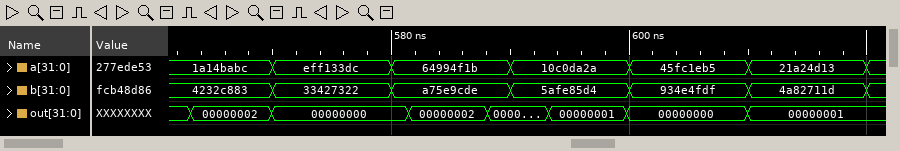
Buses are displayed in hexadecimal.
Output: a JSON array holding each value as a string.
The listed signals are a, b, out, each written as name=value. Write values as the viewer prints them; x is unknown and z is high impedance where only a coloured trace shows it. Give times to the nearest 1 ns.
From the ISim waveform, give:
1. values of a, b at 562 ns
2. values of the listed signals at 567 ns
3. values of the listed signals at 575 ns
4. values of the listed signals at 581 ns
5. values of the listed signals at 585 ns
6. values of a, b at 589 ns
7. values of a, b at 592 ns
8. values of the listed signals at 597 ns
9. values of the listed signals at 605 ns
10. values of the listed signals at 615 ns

["a=1a14babc, b=4232c883", "a=1a14babc, b=4232c883, out=00000002", "a=eff133dc, b=33427322, out=00000000", "a=64994f1b, b=a75e9cde, out=00000000", "a=64994f1b, b=a75e9cde, out=00000002", "a=64994f1b, b=a75e9cde", "a=10c0da2a, b=5afe85d4", "a=10c0da2a, b=5afe85d4, out=00000001", "a=45fc1eb5, b=934e4fdf, out=00000000", "a=21a24d13, b=4a82711d, out=00000001"]
